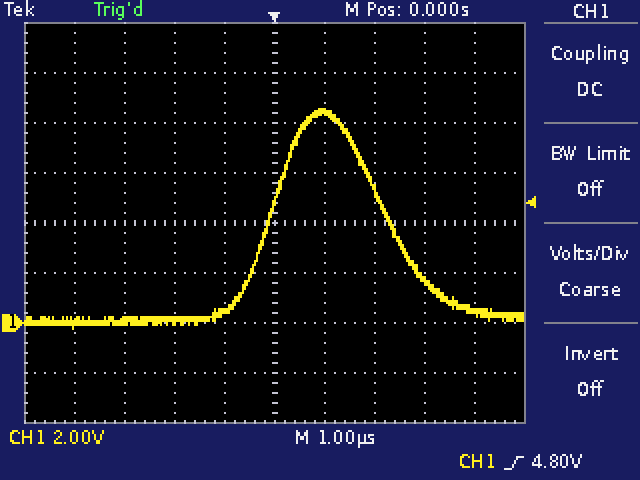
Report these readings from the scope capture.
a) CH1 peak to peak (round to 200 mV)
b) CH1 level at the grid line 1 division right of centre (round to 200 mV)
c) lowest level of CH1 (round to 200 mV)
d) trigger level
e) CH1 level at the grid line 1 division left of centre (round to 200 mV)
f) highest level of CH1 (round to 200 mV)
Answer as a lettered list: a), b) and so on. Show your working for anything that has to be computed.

a) 8.6 V − (-200 mV) = 8.8 V
b) 8.4 V
c) -200 mV
d) 4.80 V
e) 400 mV
f) 8.6 V
